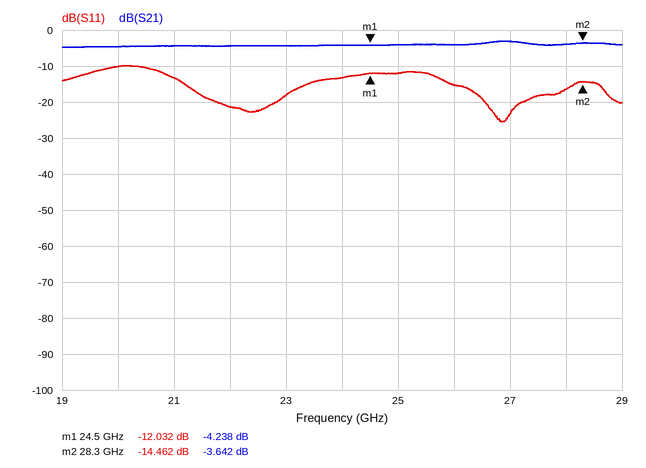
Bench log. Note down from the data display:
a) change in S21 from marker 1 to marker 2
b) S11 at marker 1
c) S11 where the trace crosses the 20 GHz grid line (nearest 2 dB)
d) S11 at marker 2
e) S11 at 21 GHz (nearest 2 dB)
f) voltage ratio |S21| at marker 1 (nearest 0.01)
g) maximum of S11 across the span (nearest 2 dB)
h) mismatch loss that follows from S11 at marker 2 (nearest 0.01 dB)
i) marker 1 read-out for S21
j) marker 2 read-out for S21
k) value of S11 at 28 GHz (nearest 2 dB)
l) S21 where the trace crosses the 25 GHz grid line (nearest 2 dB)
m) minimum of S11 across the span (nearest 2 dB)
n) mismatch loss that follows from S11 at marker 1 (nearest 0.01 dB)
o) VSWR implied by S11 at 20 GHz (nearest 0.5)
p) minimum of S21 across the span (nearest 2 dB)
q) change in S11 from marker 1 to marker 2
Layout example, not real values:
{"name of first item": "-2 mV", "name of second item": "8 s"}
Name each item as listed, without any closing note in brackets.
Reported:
{"change in S21 from marker 1 to marker 2": "0.596 dB", "S11 at marker 1": "-12.032 dB", "S11 where the trace crosses the 20 GHz grid line": "-10 dB", "S11 at marker 2": "-14.462 dB", "S11 at 21 GHz": "-14 dB", "voltage ratio |S21| at marker 1": "0.61", "maximum of S11 across the span": "-10 dB", "mismatch loss that follows from S11 at marker 2": "0.16 dB", "marker 1 read-out for S21": "-4.238 dB", "marker 2 read-out for S21": "-3.642 dB", "value of S11 at 28 GHz": "-16 dB", "S21 where the trace crosses the 25 GHz grid line": "-4 dB", "minimum of S11 across the span": "-26 dB", "mismatch loss that follows from S11 at marker 1": "0.28 dB", "VSWR implied by S11 at 20 GHz": "2.0", "minimum of S21 across the span": "-4 dB", "change in S11 from marker 1 to marker 2": "-2.430 dB"}
